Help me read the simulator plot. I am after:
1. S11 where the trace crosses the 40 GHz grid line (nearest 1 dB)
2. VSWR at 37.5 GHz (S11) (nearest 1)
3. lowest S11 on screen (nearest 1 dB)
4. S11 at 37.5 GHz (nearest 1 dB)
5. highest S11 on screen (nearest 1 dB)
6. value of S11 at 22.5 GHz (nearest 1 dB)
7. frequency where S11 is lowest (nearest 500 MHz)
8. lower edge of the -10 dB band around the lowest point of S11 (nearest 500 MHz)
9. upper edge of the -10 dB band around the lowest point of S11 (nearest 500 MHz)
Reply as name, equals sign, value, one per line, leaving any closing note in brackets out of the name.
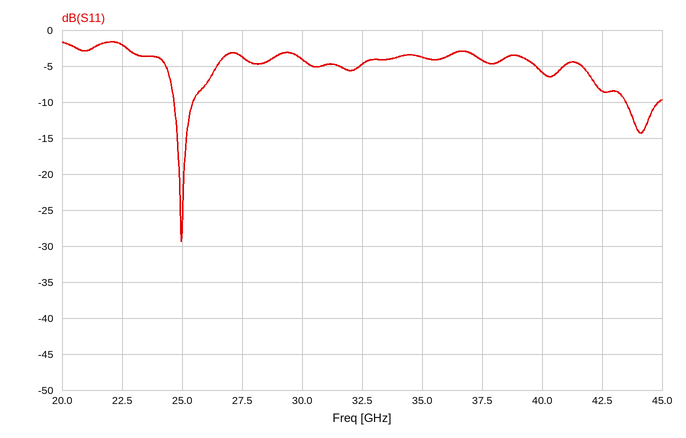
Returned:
S11 where the trace crosses the 40 GHz grid line = -6 dB
VSWR at 37.5 GHz (S11) = 4
lowest S11 on screen = -29 dB
S11 at 37.5 GHz = -4 dB
highest S11 on screen = -2 dB
value of S11 at 22.5 GHz = -2 dB
frequency where S11 is lowest = 25.0 GHz
lower edge of the -10 dB band around the lowest point of S11 = 24.5 GHz
upper edge of the -10 dB band around the lowest point of S11 = 25.5 GHz
